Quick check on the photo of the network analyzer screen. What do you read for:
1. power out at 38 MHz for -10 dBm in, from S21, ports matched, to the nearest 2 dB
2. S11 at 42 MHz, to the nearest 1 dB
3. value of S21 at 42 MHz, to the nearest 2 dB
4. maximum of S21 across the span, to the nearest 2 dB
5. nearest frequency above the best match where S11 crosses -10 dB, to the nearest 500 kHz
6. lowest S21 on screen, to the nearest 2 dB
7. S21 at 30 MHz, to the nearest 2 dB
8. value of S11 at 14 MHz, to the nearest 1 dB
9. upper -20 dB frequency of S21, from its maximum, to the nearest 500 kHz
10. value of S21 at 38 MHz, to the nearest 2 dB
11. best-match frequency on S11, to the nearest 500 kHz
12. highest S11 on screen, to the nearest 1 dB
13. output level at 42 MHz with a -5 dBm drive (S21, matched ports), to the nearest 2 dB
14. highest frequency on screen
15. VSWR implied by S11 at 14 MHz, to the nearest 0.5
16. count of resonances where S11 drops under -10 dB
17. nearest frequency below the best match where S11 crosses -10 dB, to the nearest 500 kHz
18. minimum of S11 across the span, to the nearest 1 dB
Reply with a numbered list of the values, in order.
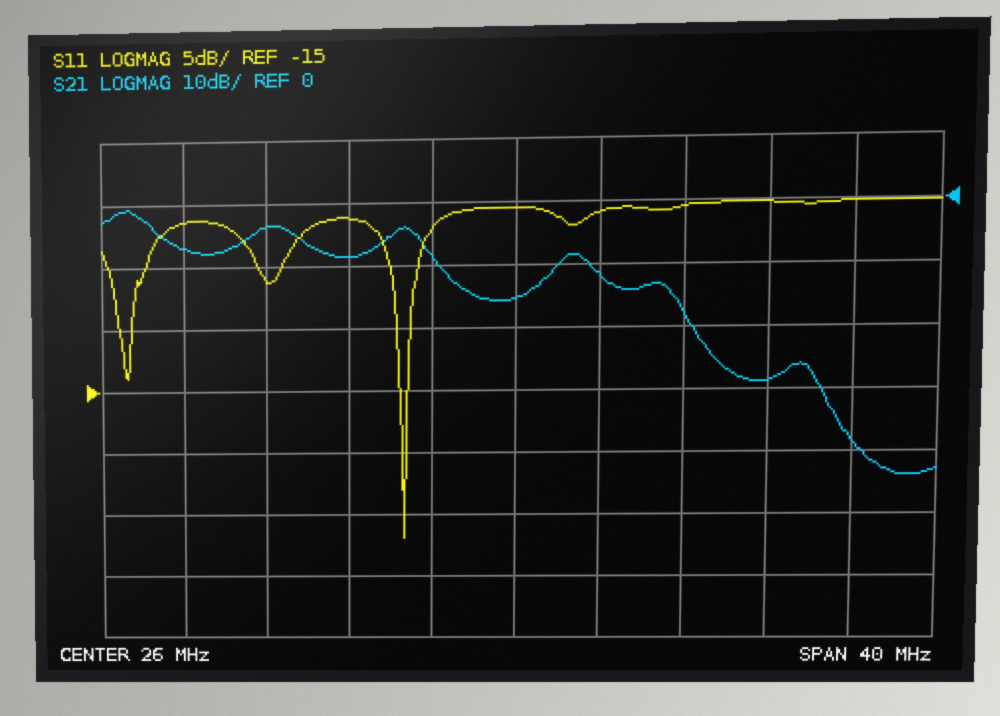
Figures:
1. -38 dBm
2. 0 dB
3. -38 dB
4. 0 dB
5. 21.0 MHz
6. -44 dB
7. -12 dB
8. -6 dB
9. 34.5 MHz
10. -28 dB
11. 20.5 MHz
12. 0 dB
13. -44 dBm
14. 46 MHz
15. 3.0
16. 2
17. 20.5 MHz
18. -27 dB
